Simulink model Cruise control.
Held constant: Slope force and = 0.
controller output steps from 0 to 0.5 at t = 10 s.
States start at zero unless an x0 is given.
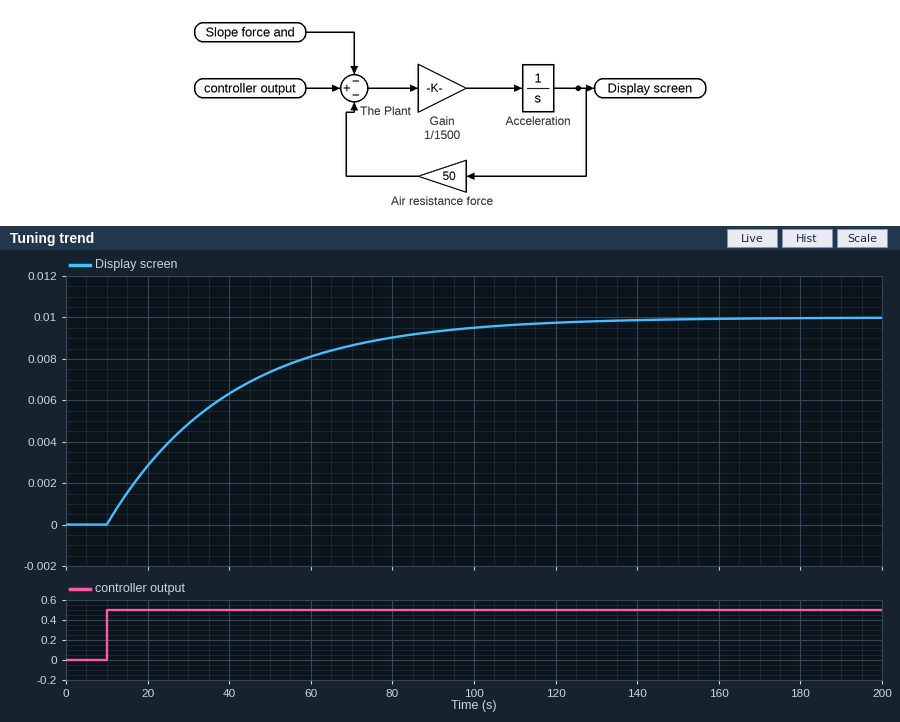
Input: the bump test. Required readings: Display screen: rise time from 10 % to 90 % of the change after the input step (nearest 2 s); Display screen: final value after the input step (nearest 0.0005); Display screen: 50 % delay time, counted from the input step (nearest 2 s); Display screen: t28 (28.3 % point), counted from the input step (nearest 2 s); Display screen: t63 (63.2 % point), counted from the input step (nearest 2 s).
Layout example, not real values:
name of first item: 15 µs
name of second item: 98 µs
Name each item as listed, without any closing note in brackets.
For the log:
Display screen: rise time from 10 % to 90 % of the change after the input step: 66 s
Display screen: final value after the input step: 0.0100
Display screen: 50 % delay time, counted from the input step: 20 s
Display screen: t28 (28.3 % point), counted from the input step: 10 s
Display screen: t63 (63.2 % point), counted from the input step: 30 s
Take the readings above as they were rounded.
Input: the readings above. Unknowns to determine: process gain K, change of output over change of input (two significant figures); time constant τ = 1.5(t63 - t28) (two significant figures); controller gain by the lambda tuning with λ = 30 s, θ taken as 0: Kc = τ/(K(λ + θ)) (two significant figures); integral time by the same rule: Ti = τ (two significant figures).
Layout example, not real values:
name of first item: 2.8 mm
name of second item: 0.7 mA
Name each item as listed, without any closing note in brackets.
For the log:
process gain K, change of output over change of input: 0.020
time constant τ = 1.5(t63 - t28): 30 s
controller gain by the lambda tuning with λ = 30 s, θ taken as 0: Kc = τ/(K(λ + θ)): 50
integral time by the same rule: Ti = τ: 30 s
